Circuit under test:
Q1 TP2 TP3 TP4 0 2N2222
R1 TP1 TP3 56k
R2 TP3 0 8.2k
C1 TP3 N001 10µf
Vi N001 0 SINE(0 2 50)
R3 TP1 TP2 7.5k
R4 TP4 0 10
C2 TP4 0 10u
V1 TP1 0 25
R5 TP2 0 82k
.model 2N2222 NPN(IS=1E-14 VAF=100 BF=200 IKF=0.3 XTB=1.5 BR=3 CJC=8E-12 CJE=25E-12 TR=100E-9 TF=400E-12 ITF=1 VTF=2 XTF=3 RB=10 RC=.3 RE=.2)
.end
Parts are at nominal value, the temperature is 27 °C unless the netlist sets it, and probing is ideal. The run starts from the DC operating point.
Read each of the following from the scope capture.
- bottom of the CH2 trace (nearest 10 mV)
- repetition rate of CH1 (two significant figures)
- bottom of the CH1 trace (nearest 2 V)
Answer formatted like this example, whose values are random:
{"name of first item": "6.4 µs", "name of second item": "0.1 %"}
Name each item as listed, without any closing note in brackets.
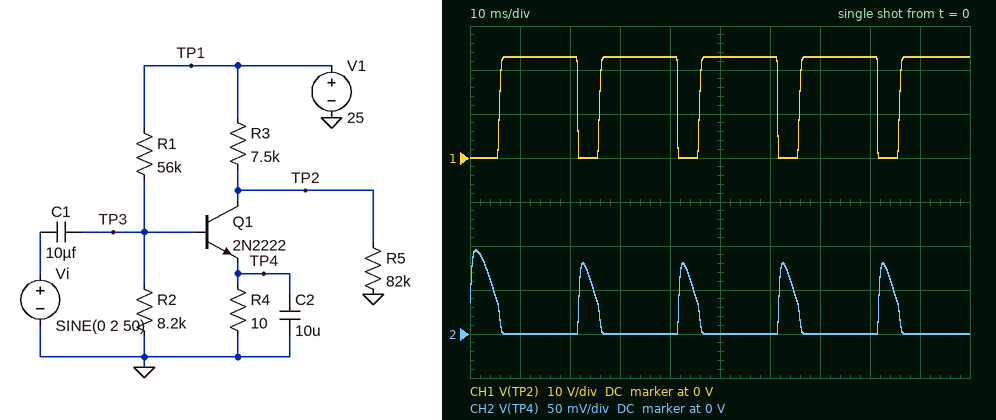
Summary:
{"bottom of the CH2 trace": "0 V", "repetition rate of CH1": "50 Hz", "bottom of the CH1 trace": "0 V"}
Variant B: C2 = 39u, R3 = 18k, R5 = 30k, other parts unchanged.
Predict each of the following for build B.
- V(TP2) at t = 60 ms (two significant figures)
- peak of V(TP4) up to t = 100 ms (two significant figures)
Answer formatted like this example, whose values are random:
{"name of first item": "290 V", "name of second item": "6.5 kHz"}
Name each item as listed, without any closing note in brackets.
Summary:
{"V(TP2) at t = 60 ms": "16 V", "peak of V(TP4) up to t = 100 ms": "72 mV"}
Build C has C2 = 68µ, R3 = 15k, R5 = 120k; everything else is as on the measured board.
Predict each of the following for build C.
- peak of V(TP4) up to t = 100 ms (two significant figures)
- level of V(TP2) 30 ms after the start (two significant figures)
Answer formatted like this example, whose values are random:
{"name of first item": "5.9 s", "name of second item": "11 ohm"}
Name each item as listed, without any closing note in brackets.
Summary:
{"peak of V(TP4) up to t = 100 ms": "71 mV", "level of V(TP2) 30 ms after the start": "22 V"}
